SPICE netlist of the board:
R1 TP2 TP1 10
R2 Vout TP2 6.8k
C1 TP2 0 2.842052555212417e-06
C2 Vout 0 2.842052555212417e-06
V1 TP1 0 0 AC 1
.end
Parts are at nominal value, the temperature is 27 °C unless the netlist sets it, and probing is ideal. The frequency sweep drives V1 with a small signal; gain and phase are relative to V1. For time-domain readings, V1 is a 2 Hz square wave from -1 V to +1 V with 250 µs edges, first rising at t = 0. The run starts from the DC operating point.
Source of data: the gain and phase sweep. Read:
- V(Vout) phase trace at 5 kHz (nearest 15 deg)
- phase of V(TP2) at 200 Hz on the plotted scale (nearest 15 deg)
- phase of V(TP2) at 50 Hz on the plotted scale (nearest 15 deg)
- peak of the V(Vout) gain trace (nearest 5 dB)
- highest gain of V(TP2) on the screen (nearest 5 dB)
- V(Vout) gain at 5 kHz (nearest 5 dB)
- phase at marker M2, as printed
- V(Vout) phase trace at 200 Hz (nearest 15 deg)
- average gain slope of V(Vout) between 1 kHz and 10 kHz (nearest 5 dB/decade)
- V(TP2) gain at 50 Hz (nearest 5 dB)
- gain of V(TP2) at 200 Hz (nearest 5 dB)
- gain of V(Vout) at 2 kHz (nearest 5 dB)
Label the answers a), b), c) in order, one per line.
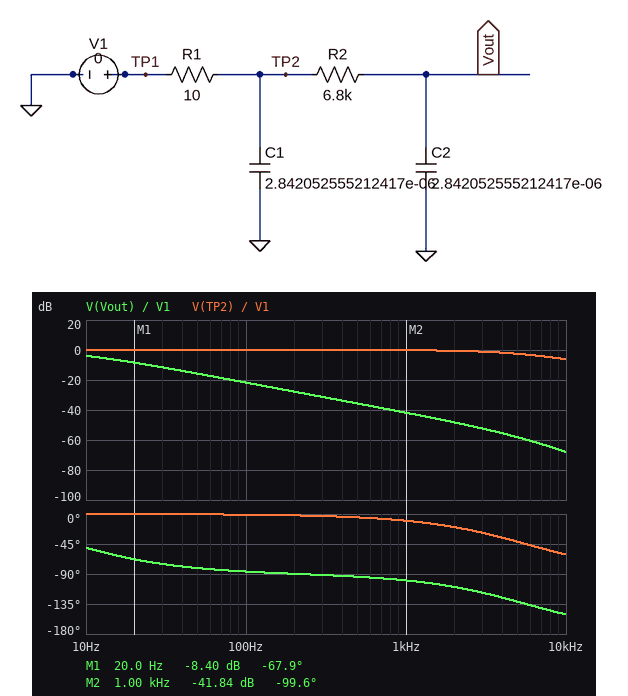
a) -135 deg
b) 0 deg
c) 0 deg
d) -5 dB
e) 0 dB
f) -60 dB
g) -99.6 deg
h) -90 deg
i) -25 dB/decade
j) 0 dB
k) 0 dB
l) -50 dB
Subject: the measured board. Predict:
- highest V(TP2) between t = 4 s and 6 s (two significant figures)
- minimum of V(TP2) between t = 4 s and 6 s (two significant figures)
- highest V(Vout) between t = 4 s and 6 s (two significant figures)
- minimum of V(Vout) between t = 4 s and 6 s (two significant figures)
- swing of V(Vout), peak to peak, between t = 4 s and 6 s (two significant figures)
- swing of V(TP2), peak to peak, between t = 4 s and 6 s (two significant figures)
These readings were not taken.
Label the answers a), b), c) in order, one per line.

a) 1.0 V
b) -1.0 V
c) 1.0 V
d) -1.0 V
e) 2.0 V
f) 2.0 V
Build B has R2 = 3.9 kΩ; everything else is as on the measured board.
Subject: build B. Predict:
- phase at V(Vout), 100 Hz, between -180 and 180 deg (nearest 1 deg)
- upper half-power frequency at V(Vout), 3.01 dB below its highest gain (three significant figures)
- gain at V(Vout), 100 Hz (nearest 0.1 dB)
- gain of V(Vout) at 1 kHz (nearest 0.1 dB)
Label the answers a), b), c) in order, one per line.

a) -83 deg
b) 14.3 Hz
c) -17.0 dB
d) -37.0 dB
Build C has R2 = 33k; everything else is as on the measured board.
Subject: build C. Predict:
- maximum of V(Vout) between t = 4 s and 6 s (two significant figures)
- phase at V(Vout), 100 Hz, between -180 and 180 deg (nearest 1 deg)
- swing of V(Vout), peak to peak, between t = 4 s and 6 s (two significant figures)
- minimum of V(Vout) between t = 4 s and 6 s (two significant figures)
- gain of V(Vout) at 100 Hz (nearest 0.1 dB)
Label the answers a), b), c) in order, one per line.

a) 870 mV
b) -90 deg
c) 1.7 V
d) -870 mV
e) -35.4 dB
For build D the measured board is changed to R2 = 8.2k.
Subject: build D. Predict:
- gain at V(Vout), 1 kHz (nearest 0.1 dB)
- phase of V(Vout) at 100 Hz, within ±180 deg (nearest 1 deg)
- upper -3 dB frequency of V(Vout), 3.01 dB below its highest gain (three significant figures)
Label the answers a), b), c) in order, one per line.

a) -43.5 dB
b) -87 deg
c) 6.82 Hz
